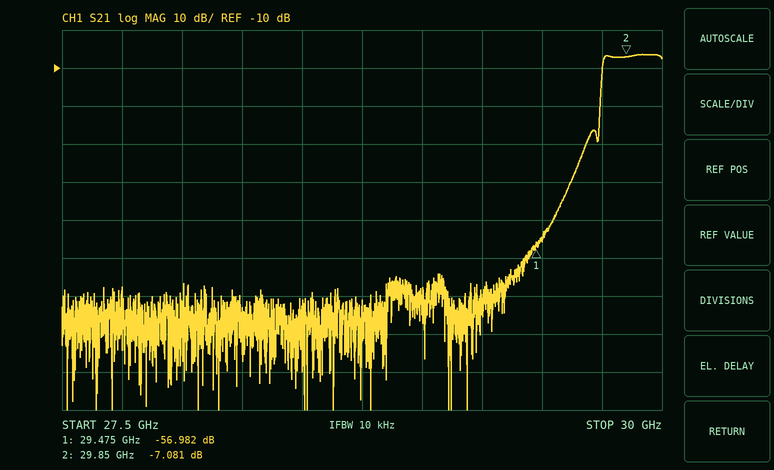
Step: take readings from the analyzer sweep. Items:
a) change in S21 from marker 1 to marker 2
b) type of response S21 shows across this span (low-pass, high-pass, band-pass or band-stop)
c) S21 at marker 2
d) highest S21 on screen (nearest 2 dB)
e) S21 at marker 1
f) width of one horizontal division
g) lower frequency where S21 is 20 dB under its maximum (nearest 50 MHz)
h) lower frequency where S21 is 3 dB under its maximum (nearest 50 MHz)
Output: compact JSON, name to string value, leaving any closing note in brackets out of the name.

{"change in S21 from marker 1 to marker 2": "49.901 dB", "type of response S21 shows across this span": "high-pass", "S21 at marker 2": "-7.081 dB", "highest S21 on screen": "-6 dB", "S21 at marker 1": "-56.982 dB", "width of one horizontal division": "250 MHz", "lower frequency where S21 is 20 dB under its maximum": "29.75 GHz", "lower frequency where S21 is 3 dB under its maximum": "29.75 GHz"}
